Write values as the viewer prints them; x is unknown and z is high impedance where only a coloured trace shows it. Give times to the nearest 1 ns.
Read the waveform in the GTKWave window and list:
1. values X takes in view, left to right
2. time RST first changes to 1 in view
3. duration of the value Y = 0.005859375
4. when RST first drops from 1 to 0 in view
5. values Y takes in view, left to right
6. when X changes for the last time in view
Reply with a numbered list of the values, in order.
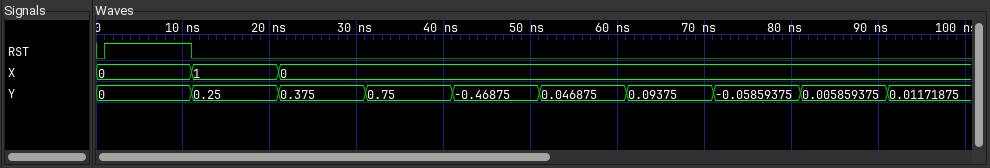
1. 0, 1, 0
2. 1 ns
3. 10 ns
4. 11 ns
5. 0, 0.25, 0.375, 0.75, -0.46875, 0.046875, 0.09375, -0.05859375, 0.005859375, 0.01171875
6. 21 ns
